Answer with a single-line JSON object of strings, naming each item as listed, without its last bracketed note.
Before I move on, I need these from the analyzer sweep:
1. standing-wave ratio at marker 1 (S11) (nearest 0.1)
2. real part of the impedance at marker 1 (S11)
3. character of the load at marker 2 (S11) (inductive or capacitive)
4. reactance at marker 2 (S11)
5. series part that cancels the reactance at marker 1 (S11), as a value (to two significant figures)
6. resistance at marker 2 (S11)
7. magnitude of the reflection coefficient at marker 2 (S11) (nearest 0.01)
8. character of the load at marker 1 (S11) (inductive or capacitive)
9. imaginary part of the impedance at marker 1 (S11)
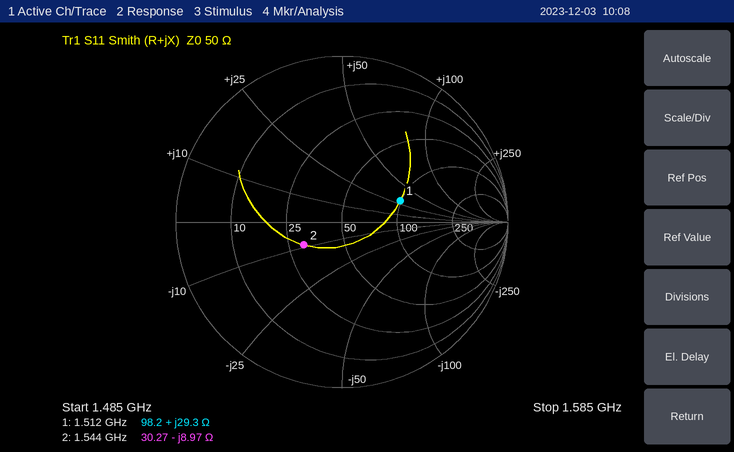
{"standing-wave ratio at marker 1 (S11)": "2.2", "real part of the impedance at marker 1": "98.2 Ω", "character of the load at marker 2 (S11)": "capacitive", "reactance at marker 2": "-8.97 Ω", "series part that cancels the reactance at marker 1 (S11), as a value": "3.6 pF", "resistance at marker 2": "30.27 Ω", "magnitude of the reflection coefficient at marker 2 (S11)": "0.27", "character of the load at marker 1 (S11)": "inductive", "imaginary part of the impedance at marker 1": "+29.3 Ω"}
